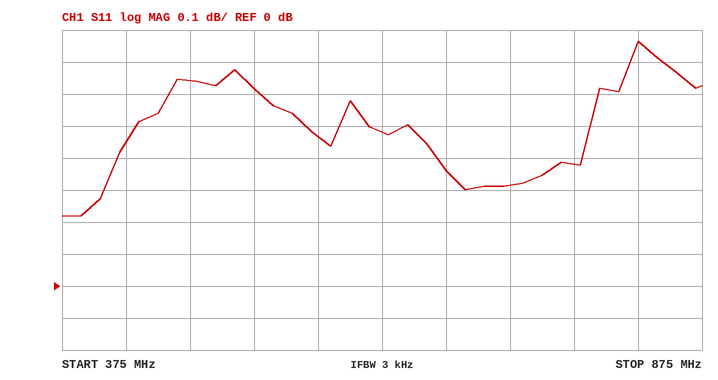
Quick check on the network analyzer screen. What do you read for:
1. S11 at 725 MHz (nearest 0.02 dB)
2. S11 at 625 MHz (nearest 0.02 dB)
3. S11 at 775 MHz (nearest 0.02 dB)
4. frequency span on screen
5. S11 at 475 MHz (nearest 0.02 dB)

0.32 dB
0.48 dB
0.38 dB
500 MHz
0.64 dB
